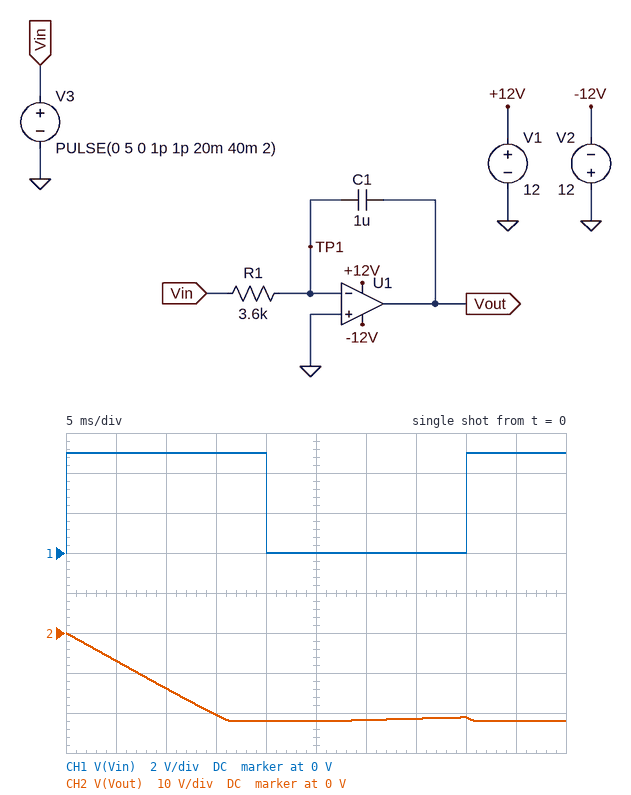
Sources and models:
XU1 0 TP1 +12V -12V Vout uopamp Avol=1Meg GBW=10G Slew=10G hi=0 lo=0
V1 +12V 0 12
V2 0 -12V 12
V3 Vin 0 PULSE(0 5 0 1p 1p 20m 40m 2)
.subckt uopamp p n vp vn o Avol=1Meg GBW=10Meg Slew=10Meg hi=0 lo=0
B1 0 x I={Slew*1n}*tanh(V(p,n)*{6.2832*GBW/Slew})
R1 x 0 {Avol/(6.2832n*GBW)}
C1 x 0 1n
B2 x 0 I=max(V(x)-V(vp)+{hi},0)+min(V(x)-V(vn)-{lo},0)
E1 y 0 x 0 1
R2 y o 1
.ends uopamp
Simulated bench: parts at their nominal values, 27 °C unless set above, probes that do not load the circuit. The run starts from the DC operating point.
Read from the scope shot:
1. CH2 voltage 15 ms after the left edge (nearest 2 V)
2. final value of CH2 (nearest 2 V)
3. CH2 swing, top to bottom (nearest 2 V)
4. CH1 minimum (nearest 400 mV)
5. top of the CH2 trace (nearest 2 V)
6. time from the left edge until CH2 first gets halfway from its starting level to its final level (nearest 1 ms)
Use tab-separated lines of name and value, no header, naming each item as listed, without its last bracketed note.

CH2 voltage 15 ms after the left edge	-20 V
final value of CH2	-22 V
CH2 swing, top to bottom	22 V
CH1 minimum	0 V
top of the CH2 trace	0 V
time from the left edge until CH2 first gets halfway from its starting level to its final level	8 ms
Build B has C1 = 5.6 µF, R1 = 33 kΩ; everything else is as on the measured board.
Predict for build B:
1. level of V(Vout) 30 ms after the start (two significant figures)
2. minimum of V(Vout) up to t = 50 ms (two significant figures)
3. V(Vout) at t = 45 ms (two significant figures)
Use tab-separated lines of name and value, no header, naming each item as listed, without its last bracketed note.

level of V(Vout) 30 ms after the start	-540 mV
minimum of V(Vout) up to t = 50 ms	-810 mV
V(Vout) at t = 45 ms	-680 mV
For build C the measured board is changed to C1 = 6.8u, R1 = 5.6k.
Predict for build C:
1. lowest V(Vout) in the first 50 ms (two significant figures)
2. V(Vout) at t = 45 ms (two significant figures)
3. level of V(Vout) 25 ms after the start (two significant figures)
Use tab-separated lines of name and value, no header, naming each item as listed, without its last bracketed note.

lowest V(Vout) in the first 50 ms	-3.9 V
V(Vout) at t = 45 ms	-3.3 V
level of V(Vout) 25 ms after the start	-2.6 V
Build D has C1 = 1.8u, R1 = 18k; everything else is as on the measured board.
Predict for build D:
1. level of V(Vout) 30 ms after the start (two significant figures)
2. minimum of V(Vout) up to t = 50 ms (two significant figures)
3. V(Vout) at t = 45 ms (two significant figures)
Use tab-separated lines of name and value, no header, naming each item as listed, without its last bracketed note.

level of V(Vout) 30 ms after the start	-3.1 V
minimum of V(Vout) up to t = 50 ms	-4.6 V
V(Vout) at t = 45 ms	-3.9 V
